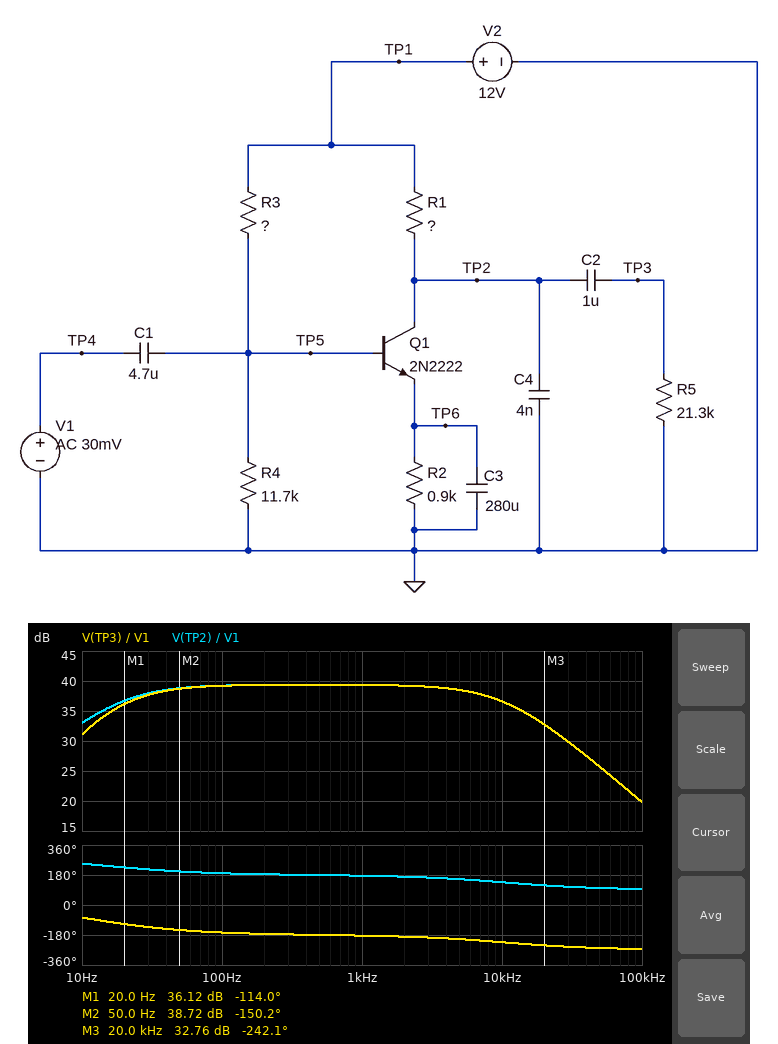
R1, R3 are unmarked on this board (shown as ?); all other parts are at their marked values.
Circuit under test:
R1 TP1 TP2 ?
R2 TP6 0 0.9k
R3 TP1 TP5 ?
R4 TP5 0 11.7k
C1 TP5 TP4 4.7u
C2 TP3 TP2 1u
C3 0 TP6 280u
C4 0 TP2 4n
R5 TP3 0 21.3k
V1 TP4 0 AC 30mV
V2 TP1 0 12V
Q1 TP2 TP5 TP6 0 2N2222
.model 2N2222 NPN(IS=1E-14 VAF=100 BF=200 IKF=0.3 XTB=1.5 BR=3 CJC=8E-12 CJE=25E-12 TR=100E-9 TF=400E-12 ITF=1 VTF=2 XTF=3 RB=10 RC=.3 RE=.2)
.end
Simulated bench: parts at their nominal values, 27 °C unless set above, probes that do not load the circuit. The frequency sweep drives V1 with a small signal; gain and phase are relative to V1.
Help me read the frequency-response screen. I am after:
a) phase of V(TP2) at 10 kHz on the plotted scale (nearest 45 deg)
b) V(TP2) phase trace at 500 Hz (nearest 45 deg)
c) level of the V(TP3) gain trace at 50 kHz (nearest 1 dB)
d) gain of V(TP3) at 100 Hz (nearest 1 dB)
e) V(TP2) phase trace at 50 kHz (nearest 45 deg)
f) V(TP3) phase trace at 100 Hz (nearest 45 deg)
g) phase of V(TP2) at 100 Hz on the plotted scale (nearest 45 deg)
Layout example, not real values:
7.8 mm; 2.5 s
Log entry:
135 deg; 180 deg; 26 dB; 39 dB; 90 deg; -180 deg; 180 deg
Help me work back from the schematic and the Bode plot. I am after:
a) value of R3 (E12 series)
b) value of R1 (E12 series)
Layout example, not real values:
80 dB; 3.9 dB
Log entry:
100 kΩ; 4.7 kΩ
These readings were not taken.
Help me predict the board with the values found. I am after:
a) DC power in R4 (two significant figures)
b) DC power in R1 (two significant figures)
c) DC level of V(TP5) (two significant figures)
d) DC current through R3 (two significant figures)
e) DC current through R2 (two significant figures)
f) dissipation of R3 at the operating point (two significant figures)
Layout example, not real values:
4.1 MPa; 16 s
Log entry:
130 µW; 2.0 mW; 1.2 V; 110 µA; 650 µA; 1.2 mW
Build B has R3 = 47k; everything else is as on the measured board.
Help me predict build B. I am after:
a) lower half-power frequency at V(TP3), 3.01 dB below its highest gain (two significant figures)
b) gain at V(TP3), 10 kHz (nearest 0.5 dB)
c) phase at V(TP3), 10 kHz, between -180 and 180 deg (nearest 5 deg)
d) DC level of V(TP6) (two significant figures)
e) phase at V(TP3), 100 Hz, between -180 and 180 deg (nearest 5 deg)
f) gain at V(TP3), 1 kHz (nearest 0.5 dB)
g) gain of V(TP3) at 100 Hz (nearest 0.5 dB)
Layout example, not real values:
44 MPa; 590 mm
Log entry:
50 Hz; 45.0 dB; 140 deg; 1.6 V; -150 deg; 48.0 dB; 47.0 dB
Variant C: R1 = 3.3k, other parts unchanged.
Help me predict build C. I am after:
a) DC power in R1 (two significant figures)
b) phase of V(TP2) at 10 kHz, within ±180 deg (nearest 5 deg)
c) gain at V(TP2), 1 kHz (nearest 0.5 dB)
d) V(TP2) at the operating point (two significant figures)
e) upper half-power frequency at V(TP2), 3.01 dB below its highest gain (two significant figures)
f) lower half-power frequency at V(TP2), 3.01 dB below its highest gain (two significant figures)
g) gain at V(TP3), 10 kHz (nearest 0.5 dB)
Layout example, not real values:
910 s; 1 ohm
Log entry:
1.4 mW; 145 deg; 37.0 dB; 9.9 V; 14 kHz; 19 Hz; 35.0 dB
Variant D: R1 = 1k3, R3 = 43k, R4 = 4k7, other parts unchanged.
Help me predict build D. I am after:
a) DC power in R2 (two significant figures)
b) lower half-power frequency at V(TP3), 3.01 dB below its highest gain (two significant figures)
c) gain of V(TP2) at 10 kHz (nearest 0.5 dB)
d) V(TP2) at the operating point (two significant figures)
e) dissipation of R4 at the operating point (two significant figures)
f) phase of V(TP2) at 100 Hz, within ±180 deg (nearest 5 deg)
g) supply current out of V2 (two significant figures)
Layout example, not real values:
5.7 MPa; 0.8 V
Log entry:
310 µW; 23 Hz; 28.5 dB; 11 V; 290 µW; -165 deg; 840 µA
